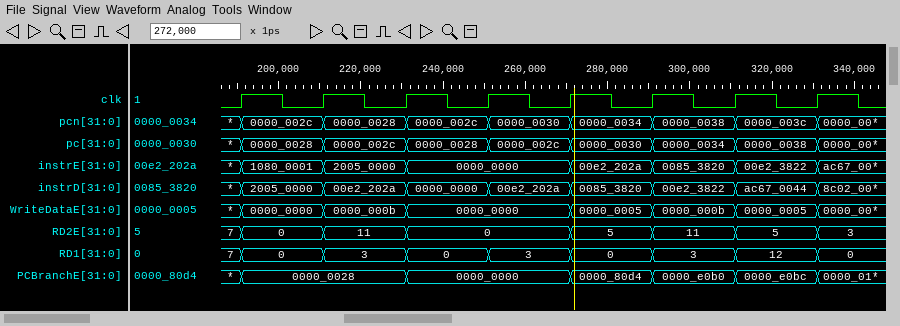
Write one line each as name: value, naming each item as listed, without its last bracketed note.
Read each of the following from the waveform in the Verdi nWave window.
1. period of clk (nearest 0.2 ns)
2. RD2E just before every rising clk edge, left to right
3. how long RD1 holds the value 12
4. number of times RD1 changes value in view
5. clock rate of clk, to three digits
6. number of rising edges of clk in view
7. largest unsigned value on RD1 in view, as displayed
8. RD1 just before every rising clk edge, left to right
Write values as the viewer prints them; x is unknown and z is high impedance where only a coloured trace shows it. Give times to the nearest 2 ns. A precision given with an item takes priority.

period of clk: 20 ns
RD2E just before every rising clk edge, left to right: 7, 0, 11, 0, 0, 5, 11, 5
how long RD1 holds the value 12: 20 ns
number of times RD1 changes value in view: 8
clock rate of clk, to three digits: 50.0 MHz
number of rising edges of clk in view: 8
largest unsigned value on RD1 in view, as displayed: 12
RD1 just before every rising clk edge, left to right: 7, 0, 3, 0, 3, 0, 3, 12
